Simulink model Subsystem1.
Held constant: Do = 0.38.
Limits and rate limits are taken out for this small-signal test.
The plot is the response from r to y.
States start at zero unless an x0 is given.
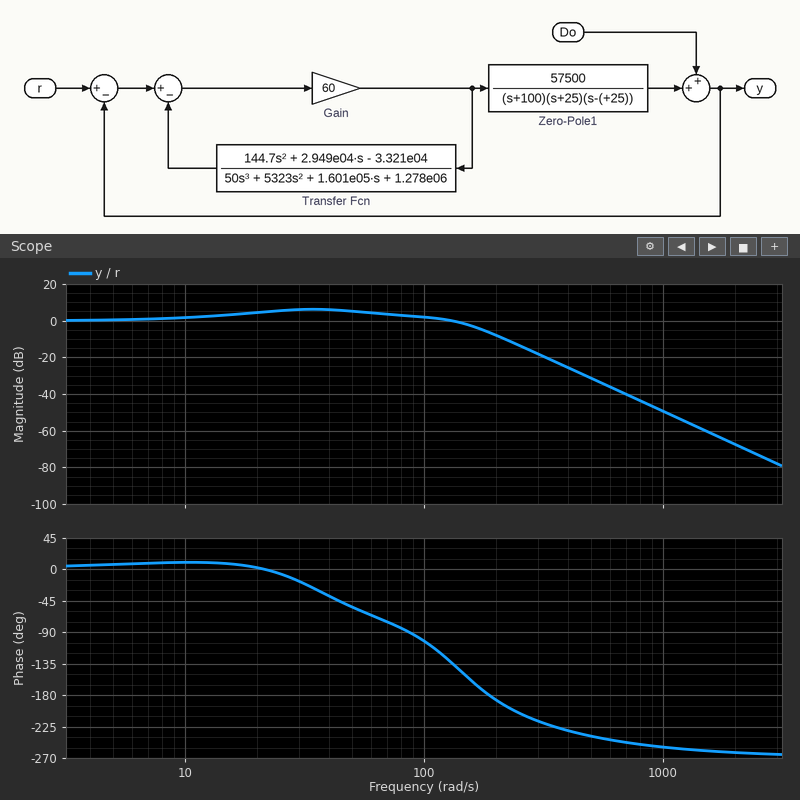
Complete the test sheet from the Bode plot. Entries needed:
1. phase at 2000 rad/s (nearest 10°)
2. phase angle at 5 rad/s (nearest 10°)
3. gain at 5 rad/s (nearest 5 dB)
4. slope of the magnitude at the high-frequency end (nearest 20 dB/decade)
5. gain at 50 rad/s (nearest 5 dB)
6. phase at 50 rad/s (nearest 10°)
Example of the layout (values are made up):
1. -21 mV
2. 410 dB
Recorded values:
1. -260°
2. 10°
3. 0 dB
4. -60 dB/decade
5. 5 dB
6. -50°
